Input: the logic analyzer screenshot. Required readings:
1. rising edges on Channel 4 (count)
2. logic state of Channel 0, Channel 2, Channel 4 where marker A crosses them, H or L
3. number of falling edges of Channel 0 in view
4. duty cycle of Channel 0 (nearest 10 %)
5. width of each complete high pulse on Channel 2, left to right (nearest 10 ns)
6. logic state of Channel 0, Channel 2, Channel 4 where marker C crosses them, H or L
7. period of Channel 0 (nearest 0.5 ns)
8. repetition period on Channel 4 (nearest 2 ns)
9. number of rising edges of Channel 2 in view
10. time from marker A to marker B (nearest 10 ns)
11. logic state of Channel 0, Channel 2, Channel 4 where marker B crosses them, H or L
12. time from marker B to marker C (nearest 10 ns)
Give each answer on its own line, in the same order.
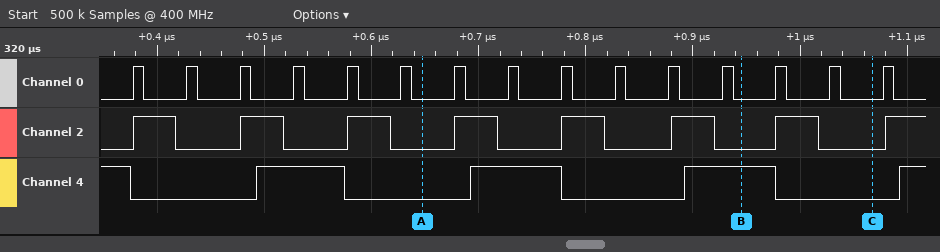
4
Channel 0=L, Channel 2=L, Channel 4=L
15
20 %
40 ns, 40 ns, 40 ns, 40 ns, 40 ns, 40 ns, 40 ns
Channel 0=L, Channel 2=L, Channel 4=L
50 ns
200 ns
8
300 ns
Channel 0=L, Channel 2=L, Channel 4=H
120 ns
